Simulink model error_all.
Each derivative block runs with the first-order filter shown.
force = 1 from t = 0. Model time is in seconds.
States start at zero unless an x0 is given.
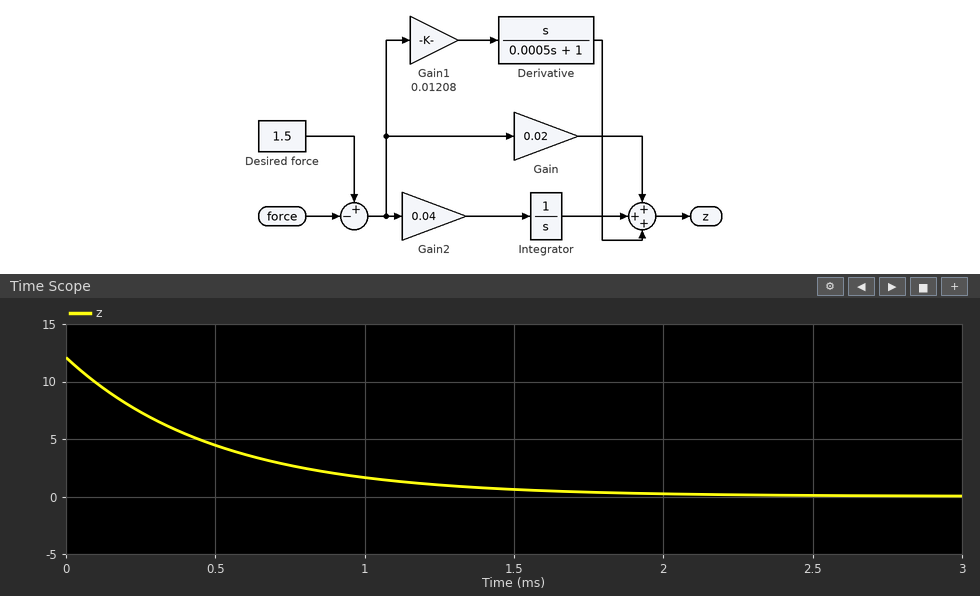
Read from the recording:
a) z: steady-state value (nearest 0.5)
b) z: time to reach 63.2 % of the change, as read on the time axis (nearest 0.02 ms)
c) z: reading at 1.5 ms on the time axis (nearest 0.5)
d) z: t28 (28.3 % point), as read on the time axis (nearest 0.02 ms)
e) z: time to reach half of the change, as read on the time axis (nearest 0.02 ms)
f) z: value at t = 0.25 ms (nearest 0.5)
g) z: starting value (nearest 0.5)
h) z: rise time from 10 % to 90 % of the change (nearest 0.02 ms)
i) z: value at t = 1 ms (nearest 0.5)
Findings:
0.0
0.50 ms
0.5
0.16 ms
0.34 ms
7.5
12.0
1.10 ms
1.5
